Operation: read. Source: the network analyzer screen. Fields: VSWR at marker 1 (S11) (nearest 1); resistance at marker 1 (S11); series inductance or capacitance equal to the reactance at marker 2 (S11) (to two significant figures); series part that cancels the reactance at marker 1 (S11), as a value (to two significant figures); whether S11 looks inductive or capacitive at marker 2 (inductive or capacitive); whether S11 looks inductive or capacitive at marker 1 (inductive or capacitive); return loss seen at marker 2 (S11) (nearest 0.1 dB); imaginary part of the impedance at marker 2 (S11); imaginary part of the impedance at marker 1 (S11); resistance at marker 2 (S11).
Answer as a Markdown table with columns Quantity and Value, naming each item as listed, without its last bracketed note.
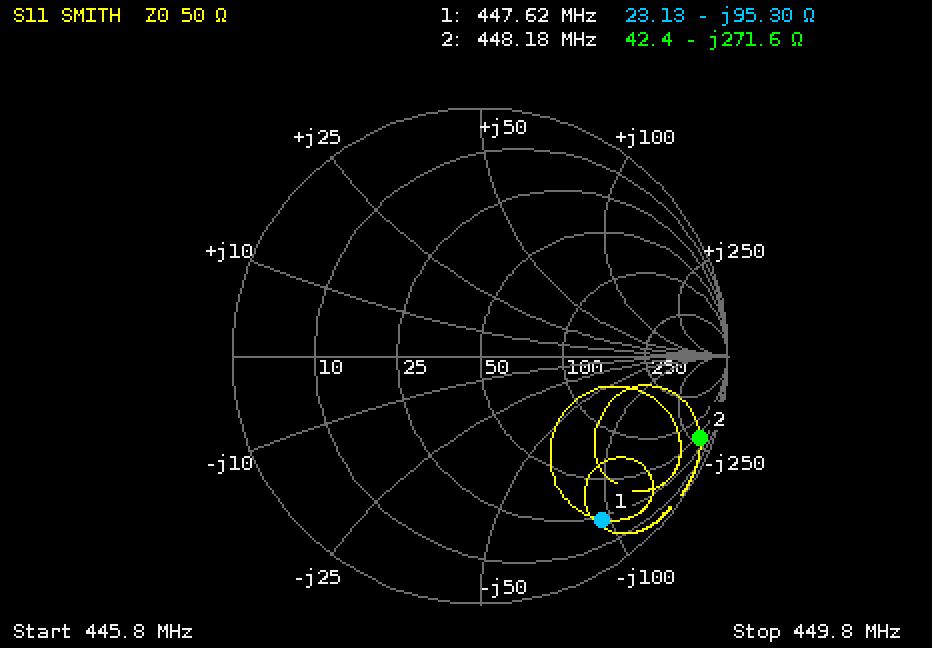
| Quantity | Value |
|---|---|
| VSWR at marker 1 (S11) | 10 |
| resistance at marker 1 | 23.13 Ω |
| series inductance or capacitance equal to the reactance at marker 2 (S11) | 1.3 pF |
| series part that cancels the reactance at marker 1 (S11), as a value | 34 nH |
| whether S11 looks inductive or capacitive at marker 2 | capacitive |
| whether S11 looks inductive or capacitive at marker 1 | capacitive |
| return loss seen at marker 2 (S11) | 0.5 dB |
| imaginary part of the impedance at marker 2 | -271.6 Ω |
| imaginary part of the impedance at marker 1 | -95.30 Ω |
| resistance at marker 2 | 42.4 Ω |
